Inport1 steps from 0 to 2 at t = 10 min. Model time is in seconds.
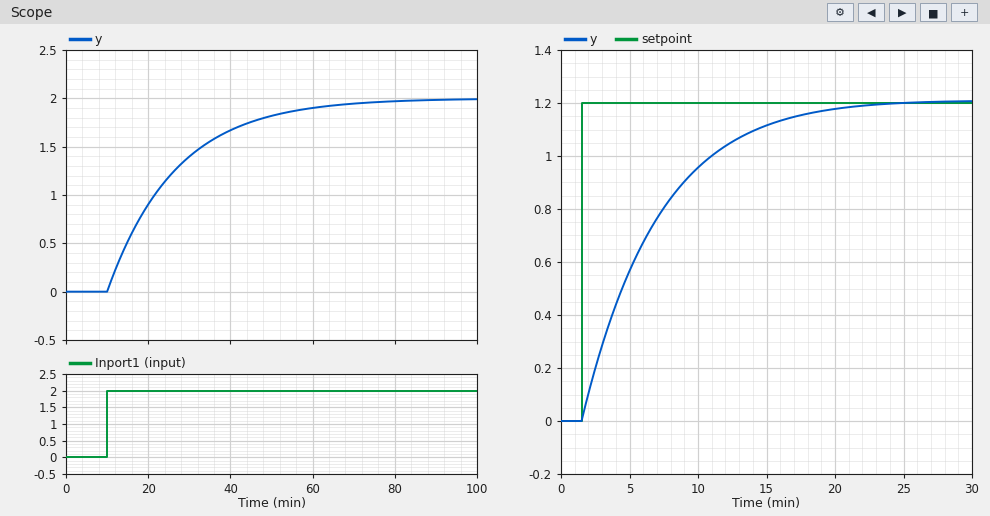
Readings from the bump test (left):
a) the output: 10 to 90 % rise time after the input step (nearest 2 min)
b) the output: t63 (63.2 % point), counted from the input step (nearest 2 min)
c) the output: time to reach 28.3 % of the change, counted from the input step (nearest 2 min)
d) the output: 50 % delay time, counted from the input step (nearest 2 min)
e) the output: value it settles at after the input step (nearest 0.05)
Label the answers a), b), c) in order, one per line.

a) 36 min
b) 16 min
c) 6 min
d) 12 min
e) 2.00
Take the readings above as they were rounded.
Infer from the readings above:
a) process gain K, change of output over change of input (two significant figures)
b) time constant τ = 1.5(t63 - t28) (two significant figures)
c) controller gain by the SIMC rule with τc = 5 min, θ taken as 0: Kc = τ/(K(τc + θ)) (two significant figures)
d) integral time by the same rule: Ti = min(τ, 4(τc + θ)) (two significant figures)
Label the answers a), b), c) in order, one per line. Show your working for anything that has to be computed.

a) (2 - 0) / 2 = 1.0
b) 1.5 × (16 - 6) = 15 min
c) 15 / (1 × (5 + 0)) = 3.0
d) min(15, 4 × (5 + 0)) = 15 min
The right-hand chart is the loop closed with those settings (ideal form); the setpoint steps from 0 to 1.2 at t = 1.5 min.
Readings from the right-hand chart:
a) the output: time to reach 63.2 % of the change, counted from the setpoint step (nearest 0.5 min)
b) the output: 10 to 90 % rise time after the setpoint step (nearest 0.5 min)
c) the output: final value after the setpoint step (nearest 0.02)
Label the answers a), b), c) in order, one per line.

a) 5.5 min
b) 11.5 min
c) 1.20
